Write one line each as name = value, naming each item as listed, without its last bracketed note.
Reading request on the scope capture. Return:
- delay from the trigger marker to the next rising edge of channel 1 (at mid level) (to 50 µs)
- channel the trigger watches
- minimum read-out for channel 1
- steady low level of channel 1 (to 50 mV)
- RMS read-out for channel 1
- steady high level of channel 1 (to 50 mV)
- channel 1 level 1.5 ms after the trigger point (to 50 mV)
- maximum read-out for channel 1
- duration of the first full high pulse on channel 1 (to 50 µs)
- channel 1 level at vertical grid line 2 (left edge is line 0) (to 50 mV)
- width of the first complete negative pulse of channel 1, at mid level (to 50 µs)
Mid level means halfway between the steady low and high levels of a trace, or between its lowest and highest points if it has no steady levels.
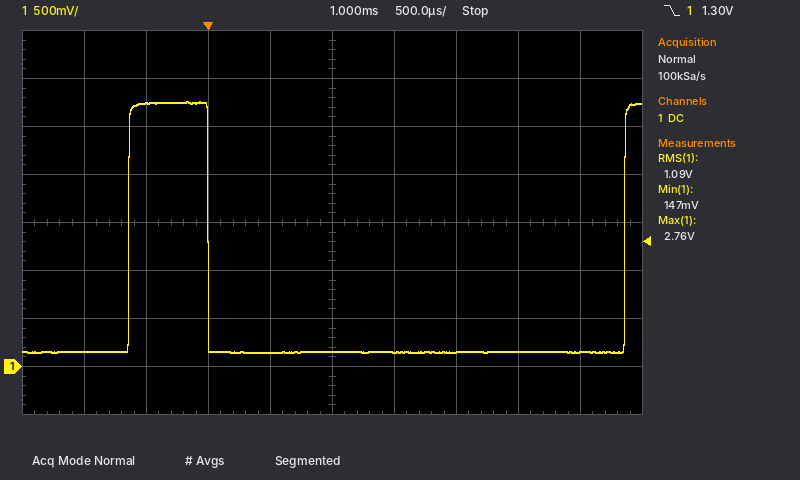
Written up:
delay from the trigger marker to the next rising edge of channel 1 (at mid level) = 3.35 ms
channel the trigger watches = channel 1
minimum read-out for channel 1 = 147 mV
steady low level of channel 1 = 150 mV
RMS read-out for channel 1 = 1.09 V
steady high level of channel 1 = 2.75 V
channel 1 level 1.5 ms after the trigger point = 150 mV
maximum read-out for channel 1 = 2.76 V
duration of the first full high pulse on channel 1 = 650 µs
channel 1 level at vertical grid line 2 (left edge is line 0) = 2.75 V
width of the first complete negative pulse of channel 1, at mid level = 3.35 ms
